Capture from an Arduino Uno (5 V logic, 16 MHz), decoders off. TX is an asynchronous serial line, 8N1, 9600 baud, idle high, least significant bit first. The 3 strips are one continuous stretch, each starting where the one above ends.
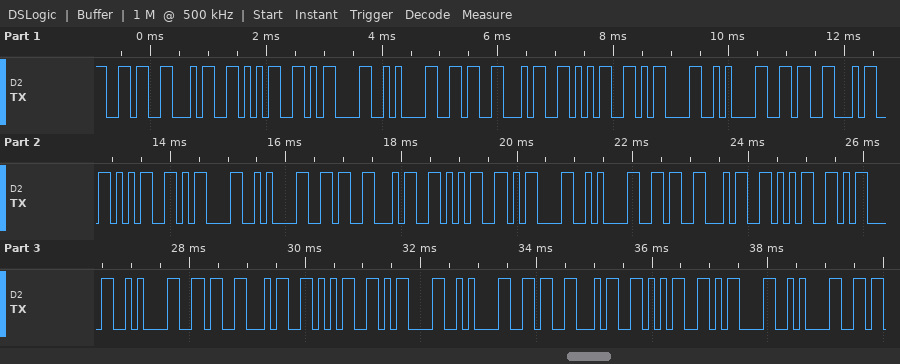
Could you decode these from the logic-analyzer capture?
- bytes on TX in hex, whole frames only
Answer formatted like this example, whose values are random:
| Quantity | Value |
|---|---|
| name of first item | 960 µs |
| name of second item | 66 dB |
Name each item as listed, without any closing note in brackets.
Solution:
| Quantity | Value |
|---|---|
| bytes on TX in hex, whole frames only | 0x36 0x34 0x35 0x0D 0x0A 0x36 0x34 0x35 0x0D 0x0A 0x36 0x34 0x35 0x0D 0x0A 0x36 0x34 0x35 0x0D 0x0A 0x36 0x34 0x35 0x0D 0x0A 0x36 0x34 0x35 0x0D 0x0A 0x36 0x34 0x35 0x0D 0x0A |
